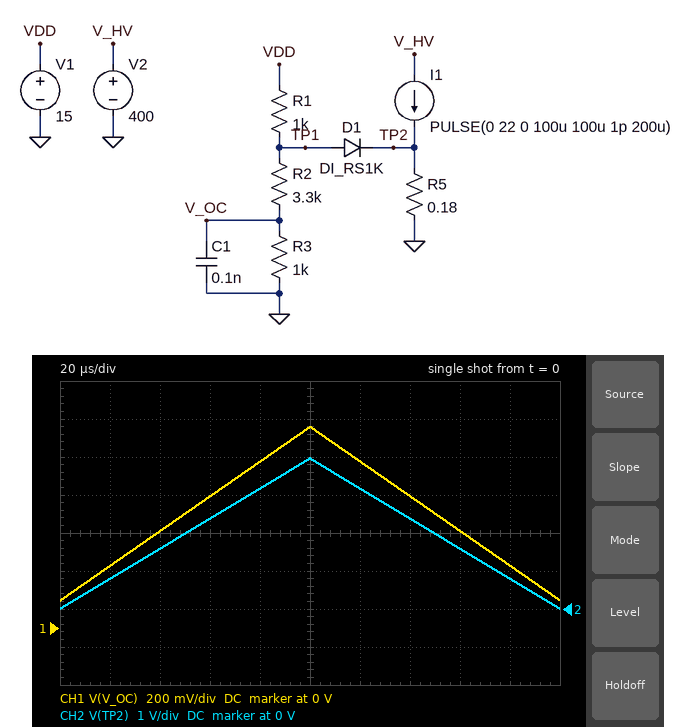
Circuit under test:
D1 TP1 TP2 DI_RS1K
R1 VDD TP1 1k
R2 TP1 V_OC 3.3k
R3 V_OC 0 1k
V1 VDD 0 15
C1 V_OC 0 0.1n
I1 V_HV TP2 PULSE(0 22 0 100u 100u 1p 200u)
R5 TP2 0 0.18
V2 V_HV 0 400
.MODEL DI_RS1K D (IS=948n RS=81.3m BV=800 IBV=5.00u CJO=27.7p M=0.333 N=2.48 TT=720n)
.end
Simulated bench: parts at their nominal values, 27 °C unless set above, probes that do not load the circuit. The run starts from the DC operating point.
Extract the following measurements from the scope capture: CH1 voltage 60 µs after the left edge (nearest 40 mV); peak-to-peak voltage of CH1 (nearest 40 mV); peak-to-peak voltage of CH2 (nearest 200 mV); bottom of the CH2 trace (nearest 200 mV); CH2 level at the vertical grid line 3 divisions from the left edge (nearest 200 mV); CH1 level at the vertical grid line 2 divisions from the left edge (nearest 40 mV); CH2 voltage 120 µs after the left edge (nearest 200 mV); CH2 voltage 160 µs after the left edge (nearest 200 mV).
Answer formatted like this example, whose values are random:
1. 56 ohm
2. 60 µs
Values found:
1. 680 mV
2. 920 mV
3. 4.0 V
4. 0 V
5. 2.4 V
6. 520 mV
7. 3.2 V
8. 1.6 V
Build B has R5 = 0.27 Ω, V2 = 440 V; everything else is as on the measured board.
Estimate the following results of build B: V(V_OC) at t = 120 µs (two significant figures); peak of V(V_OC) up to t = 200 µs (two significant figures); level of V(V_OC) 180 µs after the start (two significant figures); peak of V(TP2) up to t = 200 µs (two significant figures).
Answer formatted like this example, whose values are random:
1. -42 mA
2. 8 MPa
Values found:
1. 1.2 V
2. 1.5 V
3. 420 mV
4. 5.9 V
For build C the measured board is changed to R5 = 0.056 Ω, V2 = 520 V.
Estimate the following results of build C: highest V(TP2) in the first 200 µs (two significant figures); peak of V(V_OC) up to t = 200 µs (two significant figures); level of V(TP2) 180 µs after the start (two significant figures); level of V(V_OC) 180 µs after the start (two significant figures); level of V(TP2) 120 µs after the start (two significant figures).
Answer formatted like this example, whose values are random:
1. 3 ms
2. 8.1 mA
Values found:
1. 1.2 V
2. 430 mV
3. 250 mV
4. 200 mV
5. 990 mV
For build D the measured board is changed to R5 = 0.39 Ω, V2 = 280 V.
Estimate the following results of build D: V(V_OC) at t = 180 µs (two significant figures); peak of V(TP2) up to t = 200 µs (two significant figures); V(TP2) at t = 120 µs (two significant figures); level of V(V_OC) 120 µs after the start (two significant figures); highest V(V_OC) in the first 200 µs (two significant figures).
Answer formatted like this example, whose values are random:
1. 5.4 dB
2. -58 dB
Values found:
1. 540 mV
2. 8.6 V
3. 6.9 V
4. 1.7 V
5. 2.1 V
